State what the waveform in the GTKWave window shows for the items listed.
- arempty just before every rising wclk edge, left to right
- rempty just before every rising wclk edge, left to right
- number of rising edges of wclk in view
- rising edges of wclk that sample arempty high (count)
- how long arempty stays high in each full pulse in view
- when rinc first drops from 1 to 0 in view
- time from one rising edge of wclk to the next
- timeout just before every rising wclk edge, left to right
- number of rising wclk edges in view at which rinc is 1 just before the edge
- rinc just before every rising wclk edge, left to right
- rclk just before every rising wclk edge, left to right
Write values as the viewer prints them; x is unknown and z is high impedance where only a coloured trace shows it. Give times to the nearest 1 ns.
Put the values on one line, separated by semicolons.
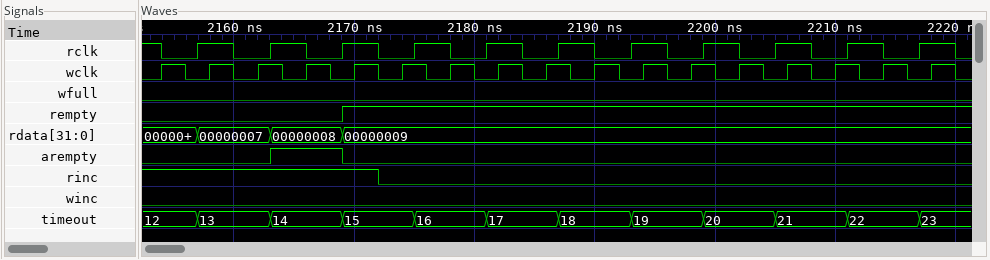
0 0 0 1 0 0 0 0 0 0 0 0 0 0 0 0 0; 0 0 0 0 1 1 1 1 1 1 1 1 1 1 1 1 1; 17; 1; 6 ns; 2172 ns; 4 ns; 12, 13, 13, 14, 15, 15, 16, 17, 17, 18, 19, 19, 20, 21, 21, 22, 23; 5; 1 1 1 1 1 0 0 0 0 0 0 0 0 0 0 0 0; 1 1 0 1 1 0 1 1 0 1 1 0 1 1 0 1 1
